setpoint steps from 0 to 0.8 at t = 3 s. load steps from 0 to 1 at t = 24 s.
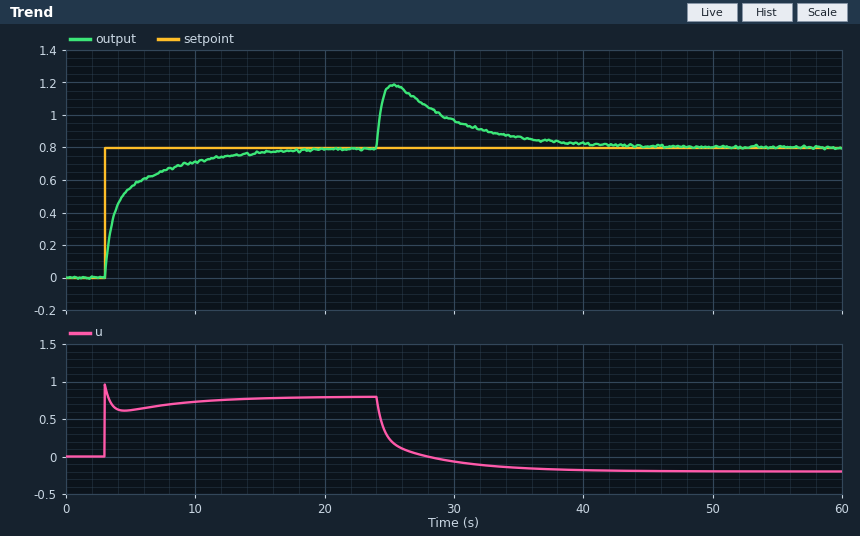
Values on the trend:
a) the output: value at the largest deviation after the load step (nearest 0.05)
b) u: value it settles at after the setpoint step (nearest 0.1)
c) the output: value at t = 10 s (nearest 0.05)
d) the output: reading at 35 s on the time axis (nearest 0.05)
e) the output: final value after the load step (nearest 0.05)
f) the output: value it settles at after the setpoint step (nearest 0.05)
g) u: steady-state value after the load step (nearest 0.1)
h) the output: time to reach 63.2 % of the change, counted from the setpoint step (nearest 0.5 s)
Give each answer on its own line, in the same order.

1.20
0.8
0.70
0.85
0.80
0.80
-0.2
1.5 s
